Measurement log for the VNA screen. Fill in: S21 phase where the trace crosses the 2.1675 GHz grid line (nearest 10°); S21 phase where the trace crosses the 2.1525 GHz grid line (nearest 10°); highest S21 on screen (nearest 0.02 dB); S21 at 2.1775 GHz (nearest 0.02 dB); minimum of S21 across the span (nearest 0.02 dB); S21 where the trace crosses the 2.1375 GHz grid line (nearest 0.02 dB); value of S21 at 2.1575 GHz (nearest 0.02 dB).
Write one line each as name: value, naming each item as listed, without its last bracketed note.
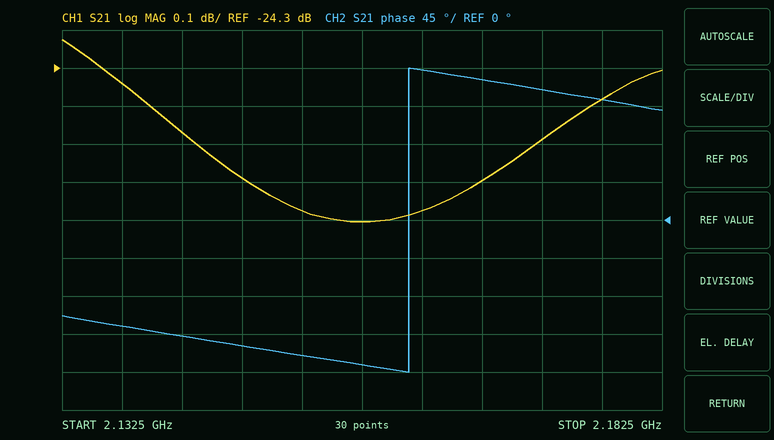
S21 phase where the trace crosses the 2.1675 GHz grid line: 170°
S21 phase where the trace crosses the 2.1525 GHz grid line: -160°
highest S21 on screen: -24.22 dB
S21 at 2.1775 GHz: -24.38 dB
minimum of S21 across the span: -24.70 dB
S21 where the trace crosses the 2.1375 GHz grid line: -24.34 dB
value of S21 at 2.1575 GHz: -24.70 dB
